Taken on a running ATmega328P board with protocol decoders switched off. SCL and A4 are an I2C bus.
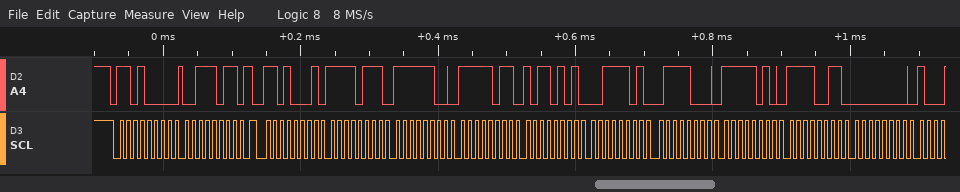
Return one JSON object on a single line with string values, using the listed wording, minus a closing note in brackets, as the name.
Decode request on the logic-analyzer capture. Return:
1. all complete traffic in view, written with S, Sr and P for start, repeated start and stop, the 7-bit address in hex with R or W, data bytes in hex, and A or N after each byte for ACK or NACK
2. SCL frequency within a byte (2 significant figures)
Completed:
{"all complete traffic in view, written with S, Sr and P for start, repeated start and stop, the 7-bit address in hex with R or W, data bytes in hex, and A or N after each byte for ACK or NACK": "S 68W A 3B A Sr 68R A F7 A FC A FB A B5 A 3D A 78 A FA A F3 A 00 A", "SCL frequency within a byte": "100 kHz"}
